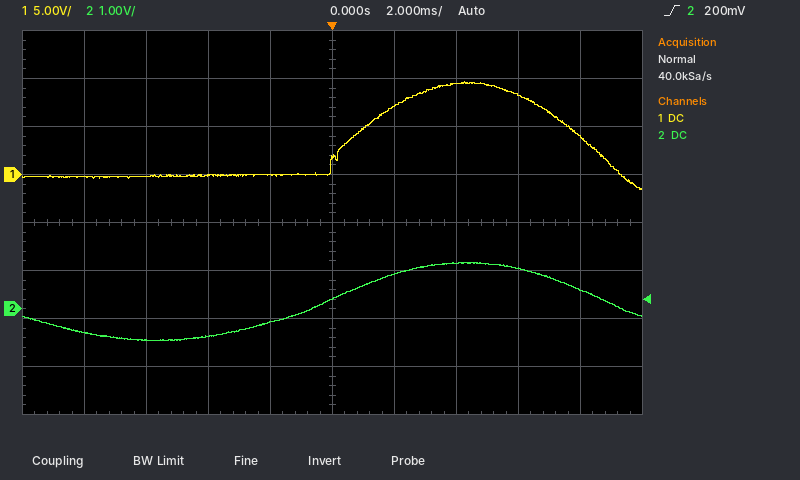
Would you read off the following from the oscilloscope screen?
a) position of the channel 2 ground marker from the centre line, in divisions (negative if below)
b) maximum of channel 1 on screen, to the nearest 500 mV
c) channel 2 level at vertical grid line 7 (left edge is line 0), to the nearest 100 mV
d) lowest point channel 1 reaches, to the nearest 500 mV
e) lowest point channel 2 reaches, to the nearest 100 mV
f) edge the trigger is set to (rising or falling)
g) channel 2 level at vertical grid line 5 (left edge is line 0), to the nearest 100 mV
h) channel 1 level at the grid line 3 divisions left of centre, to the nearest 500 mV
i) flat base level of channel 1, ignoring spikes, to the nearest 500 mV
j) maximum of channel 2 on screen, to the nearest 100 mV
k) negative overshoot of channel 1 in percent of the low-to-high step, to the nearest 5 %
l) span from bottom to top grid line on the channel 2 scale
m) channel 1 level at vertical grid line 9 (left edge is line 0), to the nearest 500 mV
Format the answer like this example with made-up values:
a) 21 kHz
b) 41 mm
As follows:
a) -1.8 div
b) 9.5 V
c) 1.0 V
d) -1.5 V
e) -700 mV
f) rising
g) 200 mV
h) 0.0 V
i) 0.0 V
j) 1.0 V
k) 15 %
l) 8 V
m) 4.0 V
